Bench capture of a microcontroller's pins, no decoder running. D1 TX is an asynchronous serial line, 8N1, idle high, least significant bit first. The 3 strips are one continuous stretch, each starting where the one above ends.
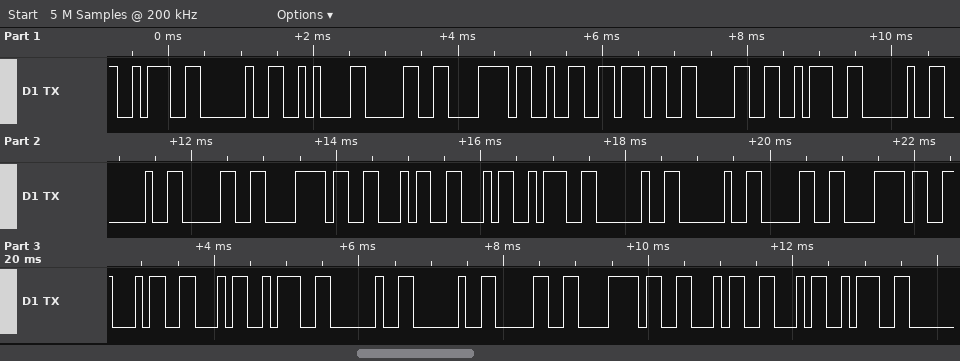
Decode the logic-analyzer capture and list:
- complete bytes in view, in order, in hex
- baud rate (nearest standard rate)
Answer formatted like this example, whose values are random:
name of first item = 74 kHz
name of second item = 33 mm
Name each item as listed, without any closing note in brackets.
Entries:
complete bytes in view, in order, in hex = 3A 20 0A 30 78 32 37 30 3A 20 20 30 78 46 46 3A 20 20 30 78 46 46 3A 20 20 30 78 46 46 3A
baud rate = 9600 baud
